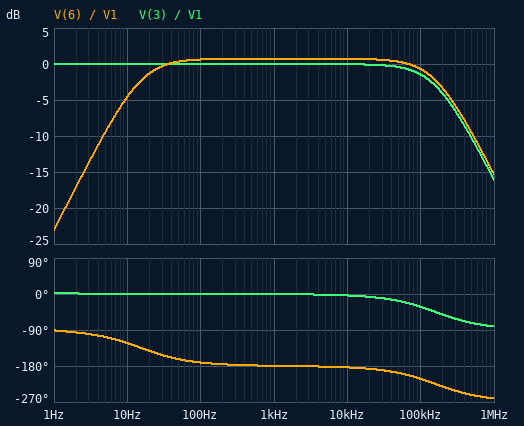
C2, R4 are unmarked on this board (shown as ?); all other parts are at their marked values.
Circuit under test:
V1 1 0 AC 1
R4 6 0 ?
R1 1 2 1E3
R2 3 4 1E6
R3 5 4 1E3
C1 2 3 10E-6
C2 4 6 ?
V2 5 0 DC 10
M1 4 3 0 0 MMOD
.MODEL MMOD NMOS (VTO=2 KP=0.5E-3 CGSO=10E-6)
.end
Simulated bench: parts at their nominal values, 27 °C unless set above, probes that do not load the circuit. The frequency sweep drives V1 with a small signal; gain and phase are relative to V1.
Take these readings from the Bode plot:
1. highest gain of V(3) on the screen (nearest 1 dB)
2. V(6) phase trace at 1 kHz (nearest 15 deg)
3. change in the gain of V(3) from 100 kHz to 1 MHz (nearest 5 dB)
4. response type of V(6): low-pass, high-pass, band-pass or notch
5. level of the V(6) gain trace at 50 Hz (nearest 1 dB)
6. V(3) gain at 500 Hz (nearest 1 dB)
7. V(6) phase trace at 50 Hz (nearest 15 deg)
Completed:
0 dB
-180 deg
-15 dB
band-pass
0 dB
0 dB
-165 deg
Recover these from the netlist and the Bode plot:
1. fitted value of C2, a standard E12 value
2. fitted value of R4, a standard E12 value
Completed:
4.7 µF
1.2 kΩ
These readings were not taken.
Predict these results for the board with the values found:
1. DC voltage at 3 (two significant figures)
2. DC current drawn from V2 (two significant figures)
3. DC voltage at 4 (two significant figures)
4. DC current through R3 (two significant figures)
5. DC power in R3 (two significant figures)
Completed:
6.0 V
4.0 mA
6.0 V
4.0 mA
16 mW
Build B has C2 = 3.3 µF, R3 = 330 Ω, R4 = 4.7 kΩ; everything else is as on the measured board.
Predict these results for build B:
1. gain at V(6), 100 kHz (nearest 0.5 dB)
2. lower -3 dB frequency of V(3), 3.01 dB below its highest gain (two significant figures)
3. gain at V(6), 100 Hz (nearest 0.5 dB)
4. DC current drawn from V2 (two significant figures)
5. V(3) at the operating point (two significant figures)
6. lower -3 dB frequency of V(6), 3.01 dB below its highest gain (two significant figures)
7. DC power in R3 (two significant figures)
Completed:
-3.0 dB
30 mHz
-1.5 dB
7.6 mA
7.5 V
9.6 Hz
19 mW
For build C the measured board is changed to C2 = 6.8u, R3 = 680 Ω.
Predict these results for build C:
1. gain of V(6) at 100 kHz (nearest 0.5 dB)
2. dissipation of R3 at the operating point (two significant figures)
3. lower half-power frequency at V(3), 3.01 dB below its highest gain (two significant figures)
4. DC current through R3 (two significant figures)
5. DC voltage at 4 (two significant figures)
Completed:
-1.5 dB
18 mW
40 mHz
5.1 mA
6.5 V
